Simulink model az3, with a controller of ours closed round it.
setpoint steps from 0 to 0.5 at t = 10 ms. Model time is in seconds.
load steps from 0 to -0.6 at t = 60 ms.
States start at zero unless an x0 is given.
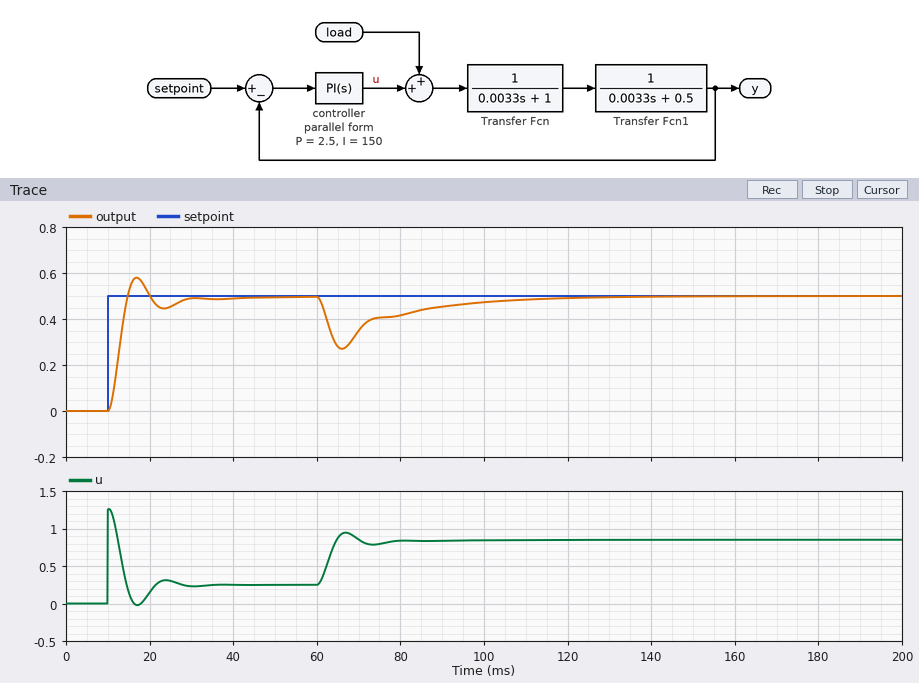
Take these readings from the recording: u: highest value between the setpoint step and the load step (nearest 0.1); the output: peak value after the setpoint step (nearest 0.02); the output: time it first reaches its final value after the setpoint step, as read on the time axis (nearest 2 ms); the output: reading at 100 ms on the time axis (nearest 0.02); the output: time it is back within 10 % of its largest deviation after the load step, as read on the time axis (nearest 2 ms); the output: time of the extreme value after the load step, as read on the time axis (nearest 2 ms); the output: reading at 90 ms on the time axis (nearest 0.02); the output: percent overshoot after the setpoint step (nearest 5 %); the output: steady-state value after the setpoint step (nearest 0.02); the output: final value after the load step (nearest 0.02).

1.3
0.58
14 ms
0.48
104 ms
66 ms
0.46
15 %
0.50
0.50
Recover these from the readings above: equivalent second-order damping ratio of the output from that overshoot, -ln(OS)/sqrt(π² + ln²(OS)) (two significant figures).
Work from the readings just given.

0.52
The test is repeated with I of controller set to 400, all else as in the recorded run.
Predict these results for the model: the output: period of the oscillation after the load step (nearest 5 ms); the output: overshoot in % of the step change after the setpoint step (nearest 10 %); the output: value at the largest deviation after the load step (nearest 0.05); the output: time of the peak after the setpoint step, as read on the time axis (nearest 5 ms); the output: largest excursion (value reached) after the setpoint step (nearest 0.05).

15 ms
40 %
0.30
15 ms
0.70
